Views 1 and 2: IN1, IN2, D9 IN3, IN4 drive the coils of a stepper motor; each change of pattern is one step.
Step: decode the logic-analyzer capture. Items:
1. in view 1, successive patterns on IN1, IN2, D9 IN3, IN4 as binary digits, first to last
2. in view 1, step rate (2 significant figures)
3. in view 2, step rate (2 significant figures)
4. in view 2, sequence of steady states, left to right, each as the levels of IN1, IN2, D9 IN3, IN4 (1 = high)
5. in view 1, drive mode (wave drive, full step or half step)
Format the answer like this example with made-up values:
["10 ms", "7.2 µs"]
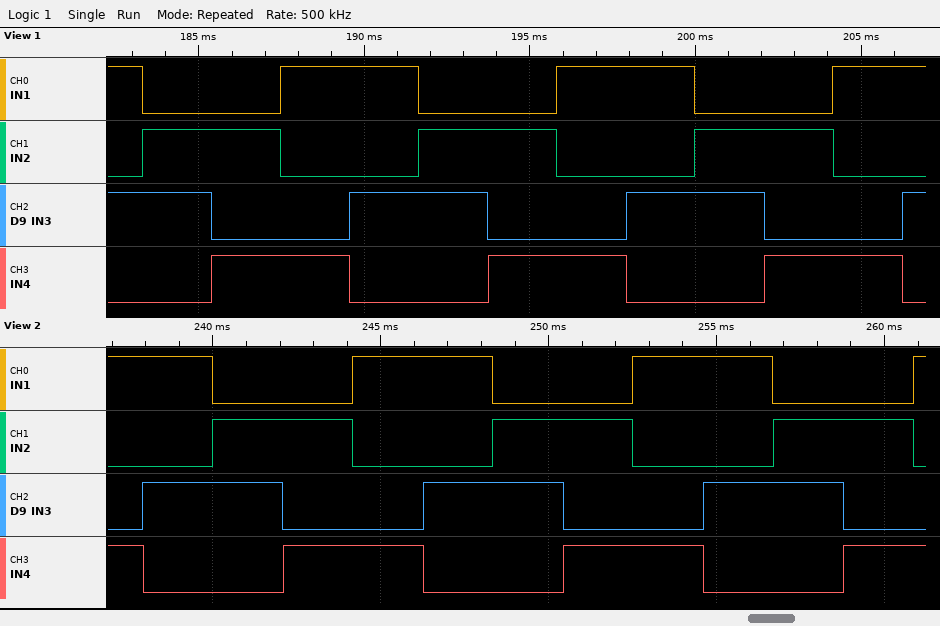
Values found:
["1010 0110 0101 1001 1010 0110 0101 1001 1010 0110 0101 1001 1010", "480 steps/s", "480 steps/s", "1001 1010 0110 0101 1001 1010 0110 0101 1001 1010 0110 0101 1001", "full step"]
